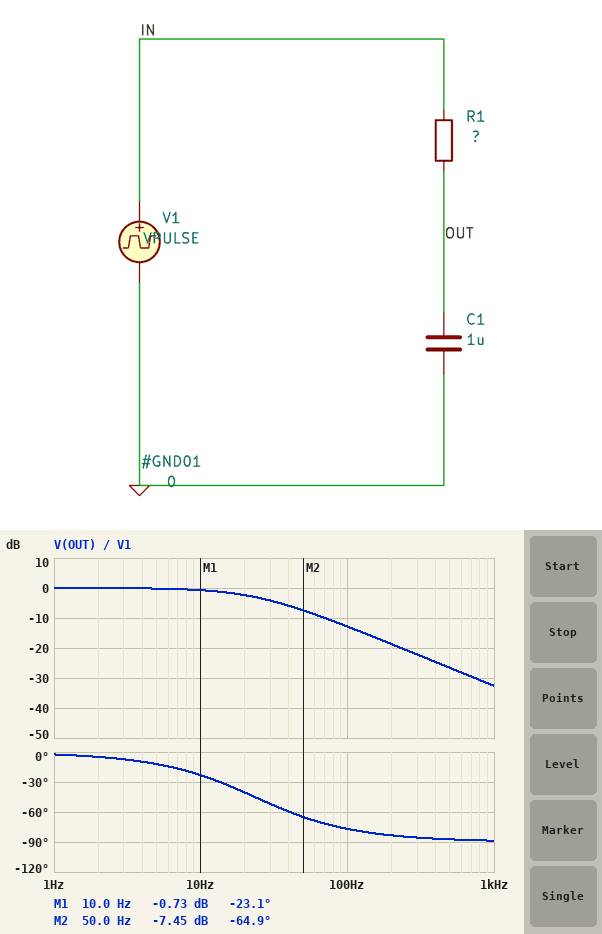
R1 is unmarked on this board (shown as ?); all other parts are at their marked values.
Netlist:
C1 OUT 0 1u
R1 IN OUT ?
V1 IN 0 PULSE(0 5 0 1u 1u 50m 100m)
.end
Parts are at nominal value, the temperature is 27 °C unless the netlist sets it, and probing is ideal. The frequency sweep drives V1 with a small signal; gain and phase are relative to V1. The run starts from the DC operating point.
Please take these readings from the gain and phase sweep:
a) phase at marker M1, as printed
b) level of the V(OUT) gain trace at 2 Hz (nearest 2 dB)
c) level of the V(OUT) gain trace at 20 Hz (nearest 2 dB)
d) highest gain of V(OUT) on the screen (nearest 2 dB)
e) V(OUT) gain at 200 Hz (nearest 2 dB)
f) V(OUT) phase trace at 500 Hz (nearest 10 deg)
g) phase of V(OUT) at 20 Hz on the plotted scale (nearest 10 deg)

-23.1 deg
0 dB
-2 dB
0 dB
-18 dB
-90 deg
-40 deg
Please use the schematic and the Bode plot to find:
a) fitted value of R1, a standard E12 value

6.8 kΩ
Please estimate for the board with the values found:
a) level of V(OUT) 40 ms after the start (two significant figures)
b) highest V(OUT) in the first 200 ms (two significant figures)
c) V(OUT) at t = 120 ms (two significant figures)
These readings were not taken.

5.0 V
5.0 V
4.7 V
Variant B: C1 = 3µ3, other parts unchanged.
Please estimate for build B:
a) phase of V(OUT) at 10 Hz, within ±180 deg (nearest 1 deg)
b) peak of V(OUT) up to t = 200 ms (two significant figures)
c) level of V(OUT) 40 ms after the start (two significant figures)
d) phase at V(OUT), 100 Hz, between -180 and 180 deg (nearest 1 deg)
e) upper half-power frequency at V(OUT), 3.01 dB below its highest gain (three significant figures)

-55 deg
4.5 V
4.2 V
-86 deg
7.09 Hz
